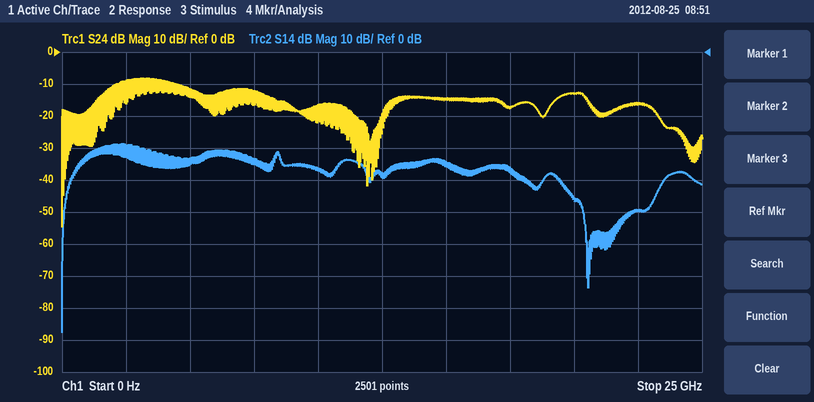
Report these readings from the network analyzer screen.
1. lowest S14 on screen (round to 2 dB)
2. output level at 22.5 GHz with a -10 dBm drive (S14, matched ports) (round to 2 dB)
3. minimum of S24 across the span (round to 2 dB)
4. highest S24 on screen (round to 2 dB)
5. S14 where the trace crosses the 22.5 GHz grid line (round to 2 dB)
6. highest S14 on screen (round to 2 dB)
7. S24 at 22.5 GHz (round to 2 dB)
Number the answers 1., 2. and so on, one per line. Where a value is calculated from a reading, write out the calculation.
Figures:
1. -88 dB
2. -10 dBm + (-50 dB) = -60 dBm
3. -54 dB
4. -8 dB
5. -50 dB
6. -28 dB
7. -16 dB
